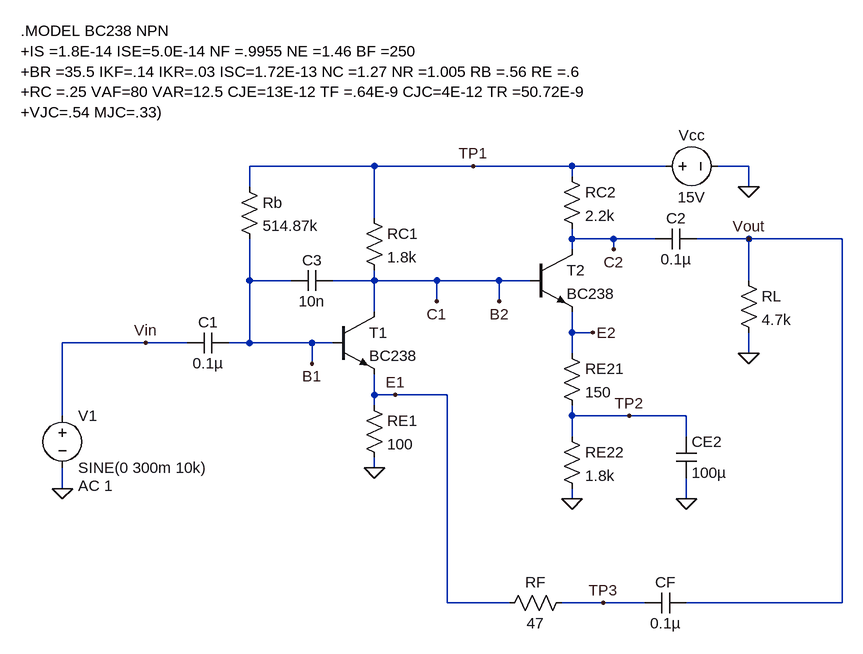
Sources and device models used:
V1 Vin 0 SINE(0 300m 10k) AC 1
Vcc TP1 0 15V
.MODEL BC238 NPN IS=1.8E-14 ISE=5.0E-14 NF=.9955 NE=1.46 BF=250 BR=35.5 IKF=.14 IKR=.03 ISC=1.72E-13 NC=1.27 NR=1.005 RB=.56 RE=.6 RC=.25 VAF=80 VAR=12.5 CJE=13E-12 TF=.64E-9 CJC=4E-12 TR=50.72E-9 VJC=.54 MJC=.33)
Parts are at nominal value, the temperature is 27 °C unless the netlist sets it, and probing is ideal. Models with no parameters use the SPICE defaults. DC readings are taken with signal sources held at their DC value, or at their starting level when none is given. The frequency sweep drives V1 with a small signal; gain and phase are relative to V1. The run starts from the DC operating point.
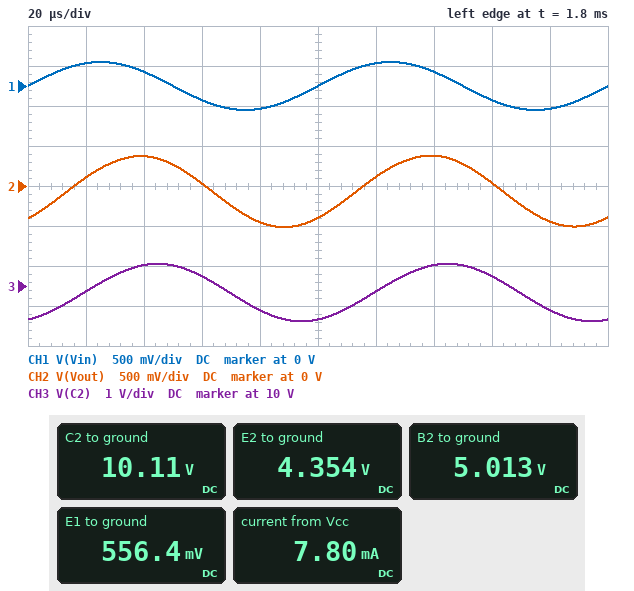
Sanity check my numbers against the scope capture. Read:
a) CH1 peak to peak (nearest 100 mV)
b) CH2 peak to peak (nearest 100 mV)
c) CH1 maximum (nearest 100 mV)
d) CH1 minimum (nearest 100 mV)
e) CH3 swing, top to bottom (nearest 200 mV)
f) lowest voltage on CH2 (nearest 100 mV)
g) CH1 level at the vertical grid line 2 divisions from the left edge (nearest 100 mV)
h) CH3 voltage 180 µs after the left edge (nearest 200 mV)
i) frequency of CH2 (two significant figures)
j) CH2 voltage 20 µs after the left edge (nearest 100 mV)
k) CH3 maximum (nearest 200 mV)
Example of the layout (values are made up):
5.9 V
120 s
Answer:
600 mV
900 mV
300 mV
-300 mV
1.4 V
-500 mV
200 mV
9.4 V
10 kHz
100 mV
10.6 V
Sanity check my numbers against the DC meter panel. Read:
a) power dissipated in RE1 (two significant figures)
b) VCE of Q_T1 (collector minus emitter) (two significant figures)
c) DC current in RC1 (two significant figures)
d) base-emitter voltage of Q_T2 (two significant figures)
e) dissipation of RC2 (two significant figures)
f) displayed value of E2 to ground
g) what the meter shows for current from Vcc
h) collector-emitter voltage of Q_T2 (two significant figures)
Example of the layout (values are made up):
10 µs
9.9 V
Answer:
3.1 mW
4.5 V
5.5 mA
660 mV
11 mW
4.354 V
7.80 mA
5.8 V
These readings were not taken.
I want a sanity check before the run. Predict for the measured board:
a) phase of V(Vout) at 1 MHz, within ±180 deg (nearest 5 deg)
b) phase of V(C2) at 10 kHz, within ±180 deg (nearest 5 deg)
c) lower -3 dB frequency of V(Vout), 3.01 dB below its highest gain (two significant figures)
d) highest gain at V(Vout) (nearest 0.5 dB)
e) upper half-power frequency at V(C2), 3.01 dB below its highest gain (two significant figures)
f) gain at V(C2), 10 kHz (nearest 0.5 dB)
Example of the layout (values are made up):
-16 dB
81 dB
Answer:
-5 deg
-70 deg
120 Hz
30.5 dB
360 Hz
7.5 dB
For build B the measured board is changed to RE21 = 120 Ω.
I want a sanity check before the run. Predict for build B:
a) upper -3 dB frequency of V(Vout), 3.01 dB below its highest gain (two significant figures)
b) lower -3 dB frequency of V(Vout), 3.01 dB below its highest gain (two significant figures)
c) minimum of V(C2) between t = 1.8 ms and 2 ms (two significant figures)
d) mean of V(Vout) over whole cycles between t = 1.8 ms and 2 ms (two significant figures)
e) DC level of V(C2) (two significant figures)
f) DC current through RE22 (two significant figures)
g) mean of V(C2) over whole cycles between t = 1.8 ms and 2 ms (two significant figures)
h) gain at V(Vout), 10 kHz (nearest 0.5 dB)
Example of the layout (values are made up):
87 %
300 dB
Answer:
390 Hz
110 Hz
8.9 V
-80 mV
10 V
2.3 mA
9.7 V
4.0 dB
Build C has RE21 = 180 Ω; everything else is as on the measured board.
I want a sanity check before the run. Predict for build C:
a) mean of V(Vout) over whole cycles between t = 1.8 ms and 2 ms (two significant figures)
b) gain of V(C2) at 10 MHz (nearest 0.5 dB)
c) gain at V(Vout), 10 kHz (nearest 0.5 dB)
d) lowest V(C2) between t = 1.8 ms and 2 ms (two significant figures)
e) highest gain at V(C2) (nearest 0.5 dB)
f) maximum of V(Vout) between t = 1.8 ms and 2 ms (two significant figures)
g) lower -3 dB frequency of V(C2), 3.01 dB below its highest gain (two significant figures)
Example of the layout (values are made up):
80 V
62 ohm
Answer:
-54 mV
-3.5 dB
3.0 dB
9.3 V
37.5 dB
370 mV
40 Hz
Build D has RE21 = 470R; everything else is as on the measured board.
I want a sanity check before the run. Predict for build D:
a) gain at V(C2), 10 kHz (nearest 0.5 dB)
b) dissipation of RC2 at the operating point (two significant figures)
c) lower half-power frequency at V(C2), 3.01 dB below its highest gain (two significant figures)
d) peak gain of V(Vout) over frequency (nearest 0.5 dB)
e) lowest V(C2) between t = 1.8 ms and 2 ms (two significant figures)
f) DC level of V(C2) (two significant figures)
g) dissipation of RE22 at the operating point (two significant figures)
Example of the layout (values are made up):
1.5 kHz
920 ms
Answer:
4.0 dB
8.0 mW
30 Hz
21.0 dB
10 V
11 V
6.6 mW
